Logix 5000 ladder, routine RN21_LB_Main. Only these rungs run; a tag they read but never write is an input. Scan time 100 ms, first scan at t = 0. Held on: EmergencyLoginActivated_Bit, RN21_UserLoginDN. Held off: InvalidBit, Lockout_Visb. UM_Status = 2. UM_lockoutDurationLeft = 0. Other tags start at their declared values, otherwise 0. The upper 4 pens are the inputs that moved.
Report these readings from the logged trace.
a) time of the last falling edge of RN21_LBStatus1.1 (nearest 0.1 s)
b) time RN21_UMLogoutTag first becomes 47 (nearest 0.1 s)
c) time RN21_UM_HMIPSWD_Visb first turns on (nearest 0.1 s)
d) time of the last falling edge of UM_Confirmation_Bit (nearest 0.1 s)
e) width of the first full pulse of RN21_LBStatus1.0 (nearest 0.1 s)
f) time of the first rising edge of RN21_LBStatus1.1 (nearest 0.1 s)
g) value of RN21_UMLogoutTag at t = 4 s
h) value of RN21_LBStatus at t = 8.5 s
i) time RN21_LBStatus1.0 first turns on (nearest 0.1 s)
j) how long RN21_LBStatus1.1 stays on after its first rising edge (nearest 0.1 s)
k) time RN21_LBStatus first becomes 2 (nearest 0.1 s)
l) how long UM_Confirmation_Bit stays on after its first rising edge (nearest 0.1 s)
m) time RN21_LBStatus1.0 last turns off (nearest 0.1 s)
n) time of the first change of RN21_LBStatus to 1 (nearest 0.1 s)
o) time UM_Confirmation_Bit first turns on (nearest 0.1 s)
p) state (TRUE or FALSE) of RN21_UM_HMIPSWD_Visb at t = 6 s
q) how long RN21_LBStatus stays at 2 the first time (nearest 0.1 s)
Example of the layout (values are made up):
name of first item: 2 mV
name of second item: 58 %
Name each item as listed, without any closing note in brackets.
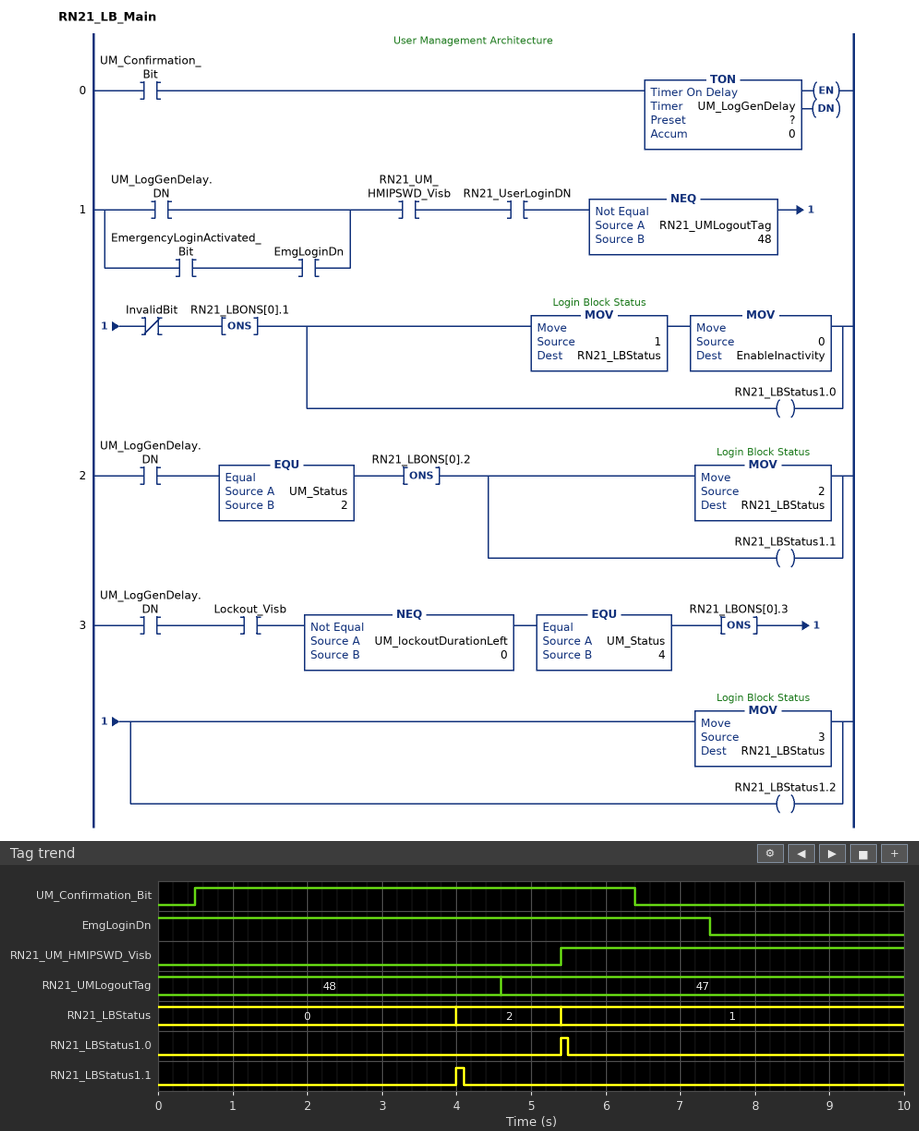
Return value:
time of the last falling edge of RN21_LBStatus1.1: 4.1 s
time RN21_UMLogoutTag first becomes 47: 4.6 s
time RN21_UM_HMIPSWD_Visb first turns on: 5.4 s
time of the last falling edge of UM_Confirmation_Bit: 6.4 s
width of the first full pulse of RN21_LBStatus1.0: 0.1 s
time of the first rising edge of RN21_LBStatus1.1: 4.0 s
value of RN21_UMLogoutTag at t = 4 s: 48
value of RN21_LBStatus at t = 8.5 s: 1
time RN21_LBStatus1.0 first turns on: 5.4 s
how long RN21_LBStatus1.1 stays on after its first rising edge: 0.1 s
time RN21_LBStatus first becomes 2: 4.0 s
how long UM_Confirmation_Bit stays on after its first rising edge: 5.9 s
time RN21_LBStatus1.0 last turns off: 5.5 s
time of the first change of RN21_LBStatus to 1: 5.4 s
time UM_Confirmation_Bit first turns on: 0.5 s
state (TRUE or FALSE) of RN21_UM_HMIPSWD_Visb at t = 6 s: TRUE
how long RN21_LBStatus stays at 2 the first time: 1.4 s
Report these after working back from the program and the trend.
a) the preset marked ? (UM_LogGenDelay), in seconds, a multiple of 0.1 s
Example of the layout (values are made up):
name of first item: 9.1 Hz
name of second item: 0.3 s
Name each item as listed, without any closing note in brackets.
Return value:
the preset marked ? (UM_LogGenDelay), in seconds, a multiple of 0.1 s: 3.5 s
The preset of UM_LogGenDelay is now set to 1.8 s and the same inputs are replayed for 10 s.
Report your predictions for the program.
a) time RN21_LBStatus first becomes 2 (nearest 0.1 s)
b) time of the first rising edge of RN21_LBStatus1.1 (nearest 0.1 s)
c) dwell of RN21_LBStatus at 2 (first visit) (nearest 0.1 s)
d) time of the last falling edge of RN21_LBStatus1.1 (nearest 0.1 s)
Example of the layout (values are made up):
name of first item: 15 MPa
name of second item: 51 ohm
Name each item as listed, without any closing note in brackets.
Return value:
time RN21_LBStatus first becomes 2: 2.3 s
time of the first rising edge of RN21_LBStatus1.1: 2.3 s
dwell of RN21_LBStatus at 2 (first visit): 3.1 s
time of the last falling edge of RN21_LBStatus1.1: 2.4 s
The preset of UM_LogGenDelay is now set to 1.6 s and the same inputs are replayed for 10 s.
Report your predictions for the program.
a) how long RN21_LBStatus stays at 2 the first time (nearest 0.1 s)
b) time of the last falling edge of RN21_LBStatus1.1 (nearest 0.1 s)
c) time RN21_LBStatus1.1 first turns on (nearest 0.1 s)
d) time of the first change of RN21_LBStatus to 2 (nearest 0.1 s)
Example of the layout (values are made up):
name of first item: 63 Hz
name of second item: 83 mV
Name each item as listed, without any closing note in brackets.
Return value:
how long RN21_LBStatus stays at 2 the first time: 3.3 s
time of the last falling edge of RN21_LBStatus1.1: 2.2 s
time RN21_LBStatus1.1 first turns on: 2.1 s
time of the first change of RN21_LBStatus to 2: 2.1 s
